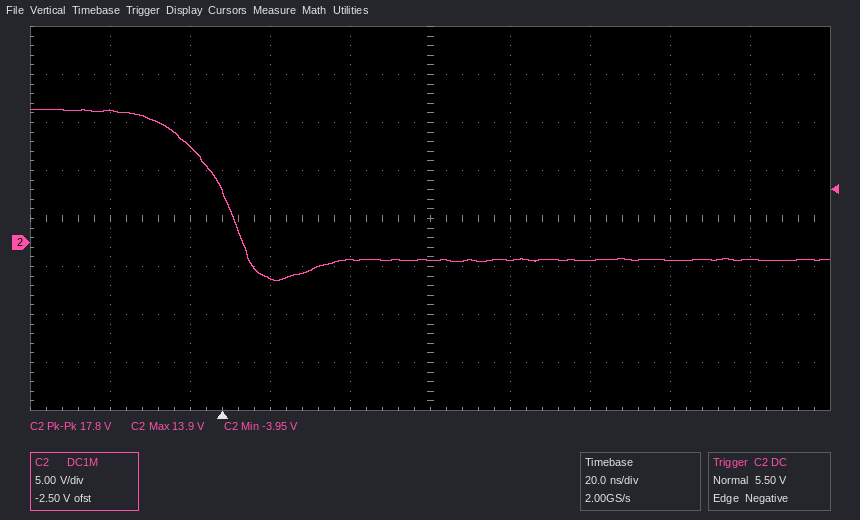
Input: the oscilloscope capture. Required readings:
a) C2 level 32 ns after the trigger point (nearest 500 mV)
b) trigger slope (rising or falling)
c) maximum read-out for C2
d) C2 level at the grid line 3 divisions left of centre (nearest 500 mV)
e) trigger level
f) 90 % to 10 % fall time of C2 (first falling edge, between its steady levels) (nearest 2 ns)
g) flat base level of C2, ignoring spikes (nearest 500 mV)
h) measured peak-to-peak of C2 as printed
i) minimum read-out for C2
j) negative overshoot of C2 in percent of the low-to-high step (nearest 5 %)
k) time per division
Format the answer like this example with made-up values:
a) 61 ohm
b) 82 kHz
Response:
a) -2.0 V
b) falling
c) 13.9 V
d) 10.0 V
e) 5.50 V
f) 20 ns
g) -2.0 V
h) 17.8 V
i) -3.95 V
j) 15 %
k) 20 ns
